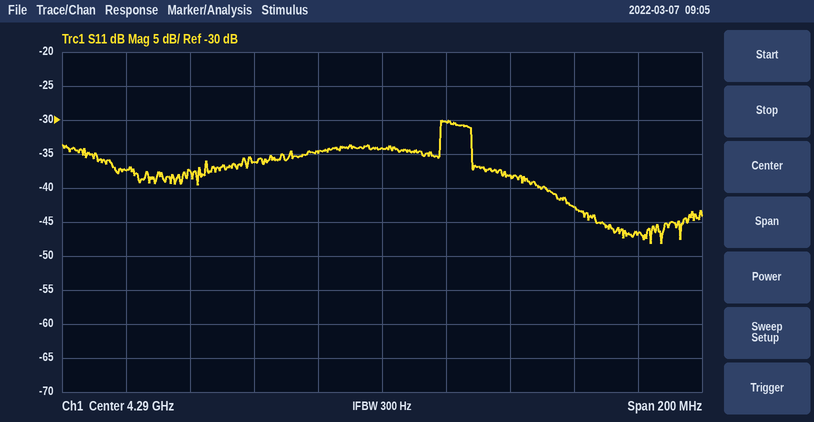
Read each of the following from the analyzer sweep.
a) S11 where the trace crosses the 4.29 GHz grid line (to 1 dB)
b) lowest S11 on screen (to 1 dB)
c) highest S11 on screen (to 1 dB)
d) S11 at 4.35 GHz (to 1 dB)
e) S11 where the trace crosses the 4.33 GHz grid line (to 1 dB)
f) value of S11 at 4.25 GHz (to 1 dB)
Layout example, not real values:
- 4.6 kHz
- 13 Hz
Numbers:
- -34 dB
- -48 dB
- -30 dB
- -43 dB
- -38 dB
- -36 dB
